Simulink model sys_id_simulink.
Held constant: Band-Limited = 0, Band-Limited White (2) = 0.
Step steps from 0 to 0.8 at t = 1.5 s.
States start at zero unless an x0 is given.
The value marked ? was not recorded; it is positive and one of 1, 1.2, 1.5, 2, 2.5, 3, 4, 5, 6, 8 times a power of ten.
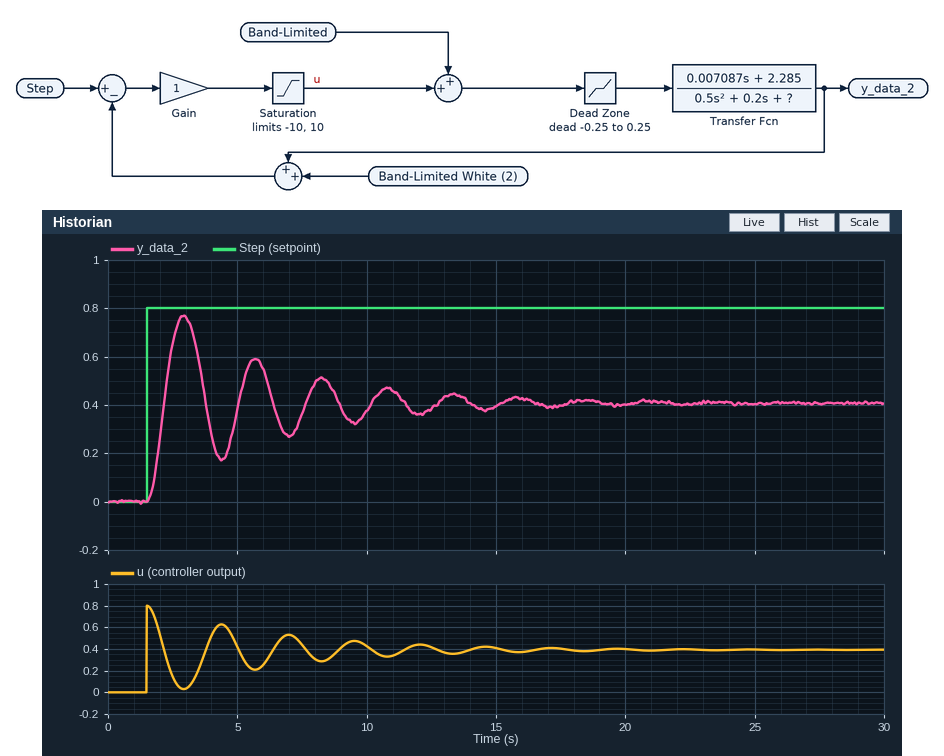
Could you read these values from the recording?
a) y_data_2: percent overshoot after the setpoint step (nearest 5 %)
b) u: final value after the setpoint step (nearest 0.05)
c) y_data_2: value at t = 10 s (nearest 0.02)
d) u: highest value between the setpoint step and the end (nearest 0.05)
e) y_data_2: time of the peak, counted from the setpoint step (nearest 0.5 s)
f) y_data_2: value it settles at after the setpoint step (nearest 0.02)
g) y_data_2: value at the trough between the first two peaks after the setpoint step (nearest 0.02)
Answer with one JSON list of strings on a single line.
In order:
["90 %", "0.40", "0.38", "0.80", "1.5 s", "0.40", "0.18"]
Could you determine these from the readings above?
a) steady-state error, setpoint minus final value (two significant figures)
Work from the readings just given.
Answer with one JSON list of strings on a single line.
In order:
["0.40"]
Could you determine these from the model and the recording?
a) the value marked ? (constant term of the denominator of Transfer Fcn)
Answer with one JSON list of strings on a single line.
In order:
["0.8"]
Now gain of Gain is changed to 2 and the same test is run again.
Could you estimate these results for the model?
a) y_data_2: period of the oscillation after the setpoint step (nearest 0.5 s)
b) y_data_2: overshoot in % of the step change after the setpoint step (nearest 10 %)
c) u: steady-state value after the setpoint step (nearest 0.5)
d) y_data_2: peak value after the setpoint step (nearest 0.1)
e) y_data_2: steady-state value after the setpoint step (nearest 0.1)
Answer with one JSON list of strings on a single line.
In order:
["2.5 s", "110 %", "0.5", "1.2", "0.6"]
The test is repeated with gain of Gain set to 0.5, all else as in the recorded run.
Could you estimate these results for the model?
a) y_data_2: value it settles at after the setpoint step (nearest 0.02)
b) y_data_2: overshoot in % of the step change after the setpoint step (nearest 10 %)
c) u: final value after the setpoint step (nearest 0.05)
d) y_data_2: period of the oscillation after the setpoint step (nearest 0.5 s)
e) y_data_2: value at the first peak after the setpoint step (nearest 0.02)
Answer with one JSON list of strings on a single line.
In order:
["0.18", "70 %", "0.30", "3.0 s", "0.30"]
